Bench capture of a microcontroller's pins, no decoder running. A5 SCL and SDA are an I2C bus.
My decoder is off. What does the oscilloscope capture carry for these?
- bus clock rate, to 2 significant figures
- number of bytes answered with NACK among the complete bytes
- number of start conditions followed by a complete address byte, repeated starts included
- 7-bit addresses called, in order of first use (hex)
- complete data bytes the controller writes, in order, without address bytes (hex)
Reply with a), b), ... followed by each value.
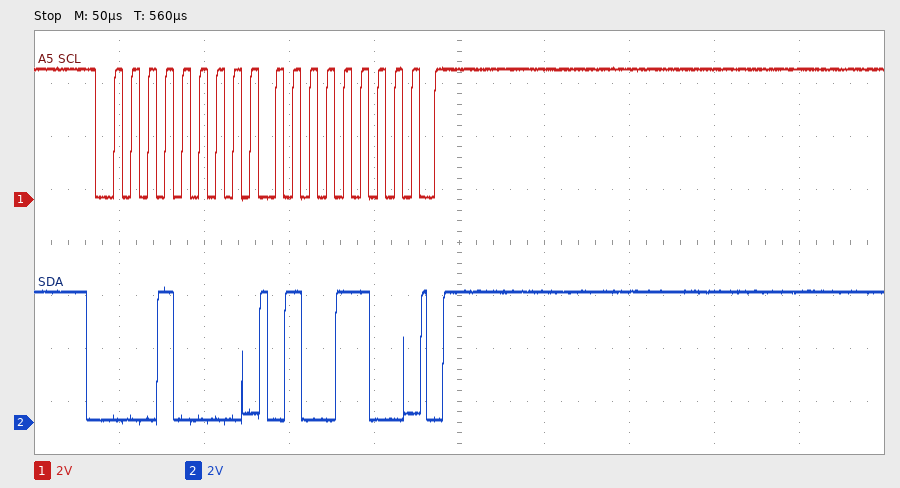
a) 100 kHz
b) 0
c) 1
d) 0x08
e) 4C
